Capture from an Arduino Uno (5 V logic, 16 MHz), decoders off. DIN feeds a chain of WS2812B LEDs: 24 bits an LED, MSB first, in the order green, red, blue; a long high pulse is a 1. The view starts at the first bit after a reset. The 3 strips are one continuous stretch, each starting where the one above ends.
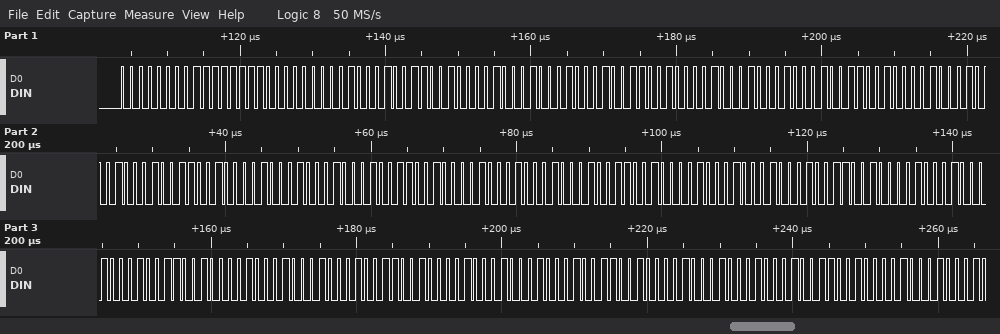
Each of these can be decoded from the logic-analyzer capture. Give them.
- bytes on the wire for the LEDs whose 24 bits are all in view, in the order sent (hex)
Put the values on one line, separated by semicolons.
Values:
00 FF 00 44 C8 44 44 C8 44 44 C8 44 44 C8 44 44 C8 44 44 C8 44 44 C8 44 44 C8 44 44 C8 44 44 C8 44 44 C8 44
